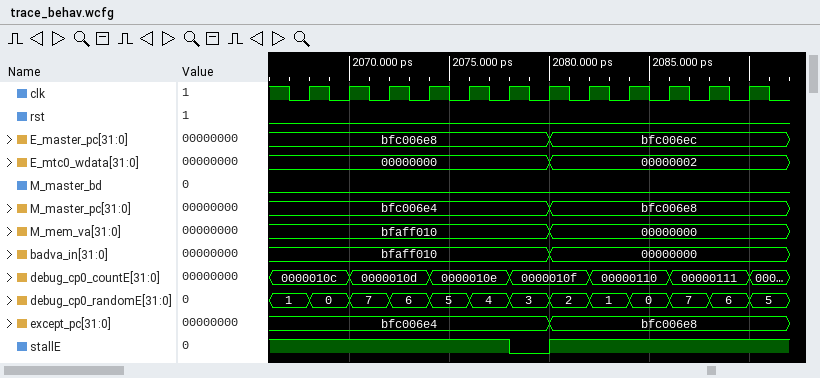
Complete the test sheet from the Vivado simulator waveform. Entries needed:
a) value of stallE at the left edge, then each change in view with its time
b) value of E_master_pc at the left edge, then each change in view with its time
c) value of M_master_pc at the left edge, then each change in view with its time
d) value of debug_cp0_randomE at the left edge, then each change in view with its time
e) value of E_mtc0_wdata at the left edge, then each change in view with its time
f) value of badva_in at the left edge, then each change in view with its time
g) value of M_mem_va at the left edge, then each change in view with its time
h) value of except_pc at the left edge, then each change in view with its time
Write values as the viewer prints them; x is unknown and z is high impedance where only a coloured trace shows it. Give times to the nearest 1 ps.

1, 0 at 2078 ps, 1 at 2080 ps
bfc006e8, bfc006ec at 2080 ps
bfc006e4, bfc006e8 at 2080 ps
1, 0 at 2068 ps, 7 at 2070 ps, 6 at 2072 ps, 5 at 2074 ps, 4 at 2076 ps, 3 at 2078 ps, 2 at 2080 ps, 1 at 2082 ps, 0 at 2084 ps, 7 at 2086 ps, 6 at 2088 ps, 5 at 2090 ps
00000000, 00000002 at 2080 ps
bfaff010, 00000000 at 2080 ps
bfaff010, 00000000 at 2080 ps
bfc006e4, bfc006e8 at 2080 ps
